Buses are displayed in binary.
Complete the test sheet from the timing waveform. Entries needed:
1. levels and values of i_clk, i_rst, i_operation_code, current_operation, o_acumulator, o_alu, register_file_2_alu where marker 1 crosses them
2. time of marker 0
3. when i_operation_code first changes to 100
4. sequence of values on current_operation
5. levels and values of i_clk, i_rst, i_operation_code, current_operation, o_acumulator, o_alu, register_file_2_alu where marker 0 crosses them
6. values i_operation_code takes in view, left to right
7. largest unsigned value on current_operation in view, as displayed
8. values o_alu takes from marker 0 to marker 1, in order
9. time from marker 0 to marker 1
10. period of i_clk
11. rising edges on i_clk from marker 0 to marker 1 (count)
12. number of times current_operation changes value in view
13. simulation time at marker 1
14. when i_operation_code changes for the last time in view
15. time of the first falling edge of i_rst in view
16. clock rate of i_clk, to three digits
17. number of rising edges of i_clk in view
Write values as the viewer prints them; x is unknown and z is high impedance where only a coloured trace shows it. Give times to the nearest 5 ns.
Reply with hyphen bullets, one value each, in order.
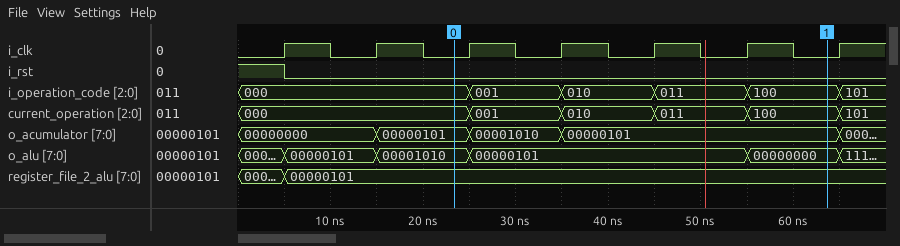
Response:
- i_clk=0, i_rst=0, i_operation_code=100, current_operation=100, o_acumulator=00000101, o_alu=00000000, register_file_2_alu=00000101
- 25 ns
- 55 ns
- 000, 001, 010, 011, 100, 101
- i_clk=0, i_rst=0, i_operation_code=000, current_operation=000, o_acumulator=00000101, o_alu=00001010, register_file_2_alu=00000101
- 000, 001, 010, 011, 100, 101
- 101
- 00001010, 00000101, 00000000
- 40 ns
- 10 ns
- 4
- 5
- 65 ns
- 65 ns
- 5 ns
- 100 MHz
- 7
